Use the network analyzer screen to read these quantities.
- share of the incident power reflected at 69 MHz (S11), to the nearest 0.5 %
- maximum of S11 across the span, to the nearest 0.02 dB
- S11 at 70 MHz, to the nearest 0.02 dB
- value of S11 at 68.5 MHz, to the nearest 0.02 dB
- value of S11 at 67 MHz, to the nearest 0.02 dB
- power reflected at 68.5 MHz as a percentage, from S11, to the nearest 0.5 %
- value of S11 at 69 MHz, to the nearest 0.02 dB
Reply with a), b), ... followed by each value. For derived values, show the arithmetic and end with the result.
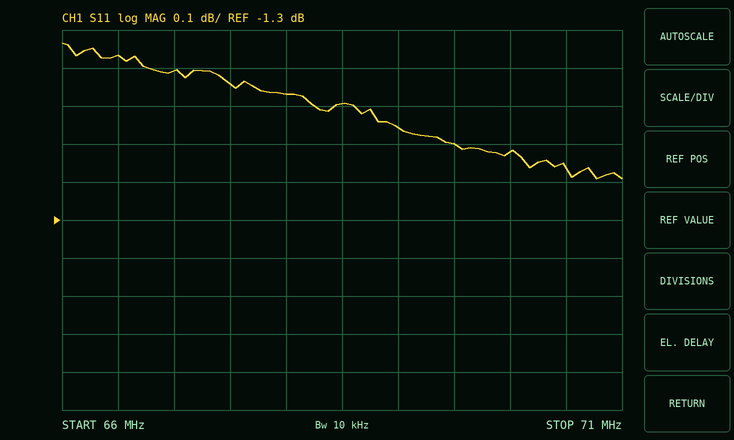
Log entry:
a) 10^(-1.06/10) ≈ 78.3 %, so 78.5 % to the nearest 0.5 %
b) -0.84 dB
c) -1.12 dB
d) -1.00 dB
e) -0.90 dB
f) 10^(-1/10) ≈ 79.4 %, so 79.5 % to the nearest 0.5 %
g) -1.06 dB
